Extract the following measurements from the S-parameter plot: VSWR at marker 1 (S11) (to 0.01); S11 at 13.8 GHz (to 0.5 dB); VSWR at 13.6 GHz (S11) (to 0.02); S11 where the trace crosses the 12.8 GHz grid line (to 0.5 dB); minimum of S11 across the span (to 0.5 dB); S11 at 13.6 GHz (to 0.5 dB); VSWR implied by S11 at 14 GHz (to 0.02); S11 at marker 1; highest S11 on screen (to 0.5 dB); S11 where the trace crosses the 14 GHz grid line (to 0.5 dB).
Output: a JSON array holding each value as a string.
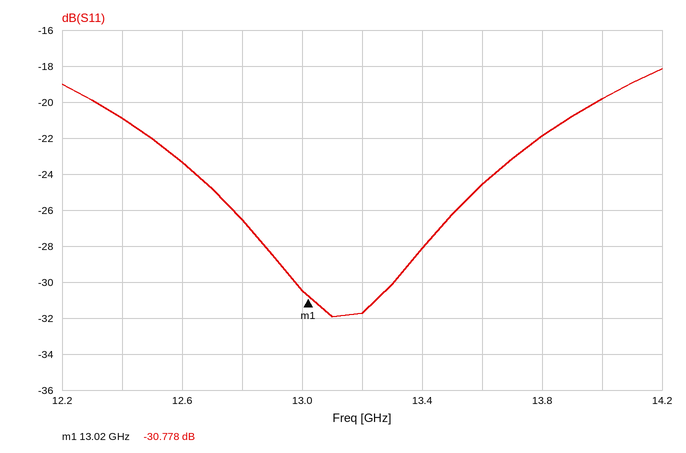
["1.06", "-22.0 dB", "1.12", "-26.5 dB", "-32.0 dB", "-24.5 dB", "1.22", "-30.778 dB", "-18.0 dB", "-20.0 dB"]
